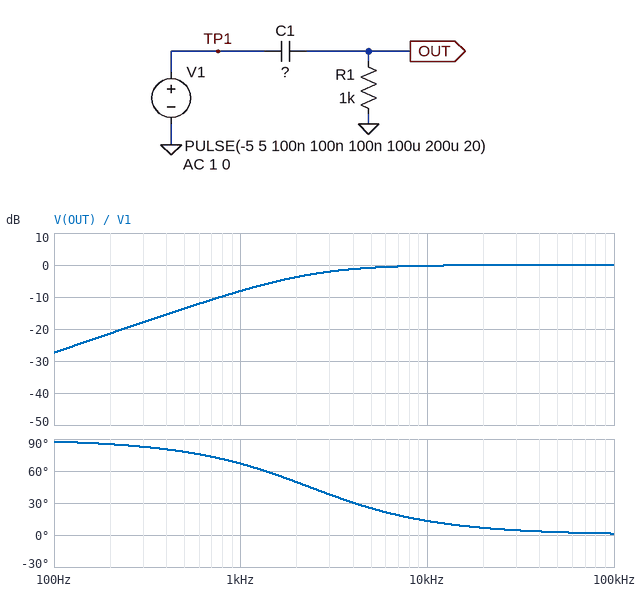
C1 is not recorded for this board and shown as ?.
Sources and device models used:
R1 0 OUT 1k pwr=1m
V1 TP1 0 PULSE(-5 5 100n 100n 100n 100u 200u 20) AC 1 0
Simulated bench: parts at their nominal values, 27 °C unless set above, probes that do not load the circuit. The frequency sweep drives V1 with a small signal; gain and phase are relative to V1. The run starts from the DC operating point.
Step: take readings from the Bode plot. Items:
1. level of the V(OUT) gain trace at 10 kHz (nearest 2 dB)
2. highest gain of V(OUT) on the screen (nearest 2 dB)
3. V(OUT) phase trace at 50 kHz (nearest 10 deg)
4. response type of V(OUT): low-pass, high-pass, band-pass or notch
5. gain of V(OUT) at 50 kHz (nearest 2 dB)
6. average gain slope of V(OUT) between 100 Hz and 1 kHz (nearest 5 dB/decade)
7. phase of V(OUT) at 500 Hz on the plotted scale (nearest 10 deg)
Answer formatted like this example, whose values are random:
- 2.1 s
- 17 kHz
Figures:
- 0 dB
- 0 dB
- 0 deg
- high-pass
- 0 dB
- 20 dB/decade
- 80 deg
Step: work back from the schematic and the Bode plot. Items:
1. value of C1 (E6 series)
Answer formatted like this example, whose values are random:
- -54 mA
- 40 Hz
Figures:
- 68 nF
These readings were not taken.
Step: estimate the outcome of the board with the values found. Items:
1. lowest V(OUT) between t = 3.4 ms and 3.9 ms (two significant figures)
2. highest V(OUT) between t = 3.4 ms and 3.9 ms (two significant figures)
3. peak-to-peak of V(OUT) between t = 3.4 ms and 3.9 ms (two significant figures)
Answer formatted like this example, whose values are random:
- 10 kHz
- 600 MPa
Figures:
- -8.1 V
- 8.1 V
- 16 V
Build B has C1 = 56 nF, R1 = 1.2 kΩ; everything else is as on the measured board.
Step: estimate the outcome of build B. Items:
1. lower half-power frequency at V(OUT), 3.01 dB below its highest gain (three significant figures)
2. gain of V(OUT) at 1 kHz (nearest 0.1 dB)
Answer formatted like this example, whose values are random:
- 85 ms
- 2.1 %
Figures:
- 2.37 kHz
- -8.2 dB
